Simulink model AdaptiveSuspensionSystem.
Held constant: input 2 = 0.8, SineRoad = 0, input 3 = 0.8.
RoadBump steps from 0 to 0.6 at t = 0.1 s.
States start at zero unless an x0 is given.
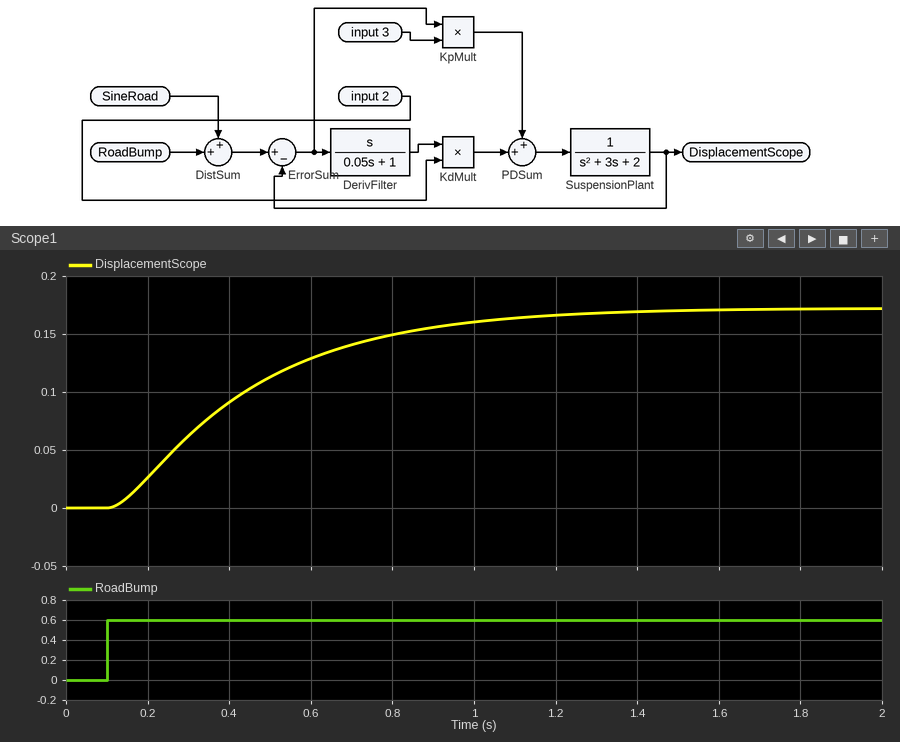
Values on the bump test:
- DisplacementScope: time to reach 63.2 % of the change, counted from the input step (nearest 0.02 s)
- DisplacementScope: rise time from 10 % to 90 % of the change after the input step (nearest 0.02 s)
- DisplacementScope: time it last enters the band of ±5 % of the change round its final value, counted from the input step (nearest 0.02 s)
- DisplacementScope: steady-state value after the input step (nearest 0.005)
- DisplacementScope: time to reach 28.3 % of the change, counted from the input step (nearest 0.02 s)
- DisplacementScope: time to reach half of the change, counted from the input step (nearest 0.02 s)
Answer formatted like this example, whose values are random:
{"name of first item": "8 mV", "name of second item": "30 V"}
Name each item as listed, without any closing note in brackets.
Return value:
{"DisplacementScope: time to reach 63.2 % of the change, counted from the input step": "0.38 s", "DisplacementScope: rise time from 10 % to 90 % of the change after the input step": "0.70 s", "DisplacementScope: time it last enters the band of ±5 % of the change round its final value, counted from the input step": "0.98 s", "DisplacementScope: steady-state value after the input step": "0.170", "DisplacementScope: time to reach 28.3 % of the change, counted from the input step": "0.16 s", "DisplacementScope: time to reach half of the change, counted from the input step": "0.28 s"}
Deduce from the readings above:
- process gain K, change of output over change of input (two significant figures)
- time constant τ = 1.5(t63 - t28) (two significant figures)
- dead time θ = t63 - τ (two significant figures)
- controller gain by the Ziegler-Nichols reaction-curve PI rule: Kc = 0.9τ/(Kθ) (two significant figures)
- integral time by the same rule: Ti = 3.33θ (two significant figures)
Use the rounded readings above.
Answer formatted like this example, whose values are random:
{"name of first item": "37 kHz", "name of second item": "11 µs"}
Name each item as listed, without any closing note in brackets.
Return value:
{"process gain K, change of output over change of input": "0.28", "time constant τ = 1.5(t63 - t28)": "0.33 s", "dead time θ = t63 - τ": "0.050 s", "controller gain by the Ziegler-Nichols reaction-curve PI rule: Kc = 0.9τ/(Kθ)": "21", "integral time by the same rule: Ti = 3.33θ": "0.17 s"}
